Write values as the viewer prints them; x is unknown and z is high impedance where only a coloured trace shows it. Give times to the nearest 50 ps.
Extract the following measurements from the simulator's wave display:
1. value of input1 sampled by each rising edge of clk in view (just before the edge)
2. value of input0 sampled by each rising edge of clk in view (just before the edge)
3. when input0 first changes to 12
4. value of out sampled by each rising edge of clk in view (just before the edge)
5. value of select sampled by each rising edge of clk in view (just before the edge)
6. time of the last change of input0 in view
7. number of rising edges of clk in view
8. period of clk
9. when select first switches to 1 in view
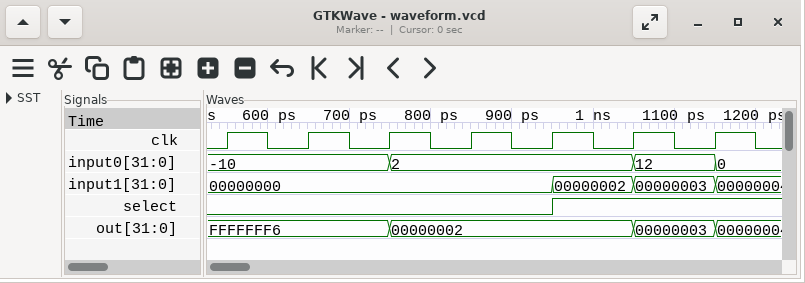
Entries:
00000000, 00000000, 00000000, 00000000, 00000000, 00000002, 00000003
-10, -10, -10, 2, 2, 2, 12
1050 ps
FFFFFFF6, FFFFFFF6, FFFFFFF6, 00000002, 00000002, 00000002, 00000003
0 0 0 0 0 1 1
1150 ps
7
100 ps
950 ps
